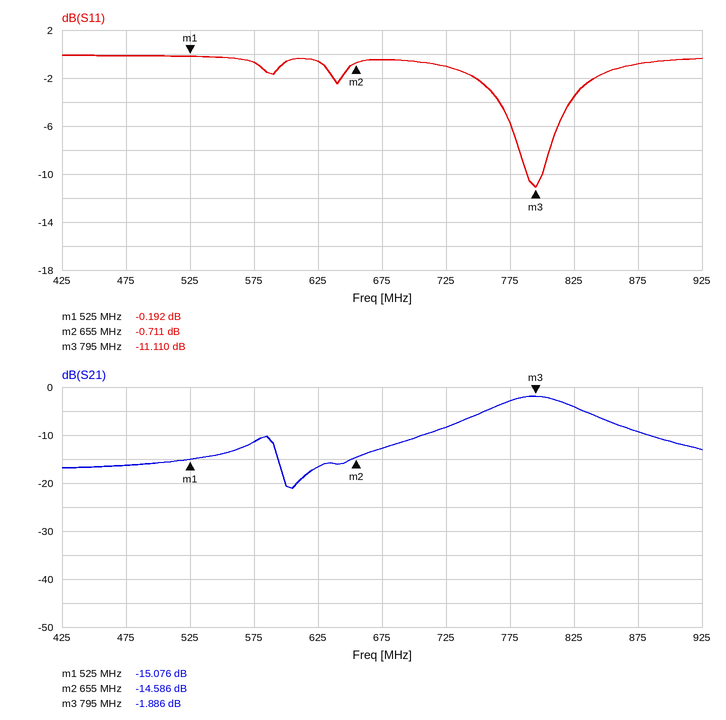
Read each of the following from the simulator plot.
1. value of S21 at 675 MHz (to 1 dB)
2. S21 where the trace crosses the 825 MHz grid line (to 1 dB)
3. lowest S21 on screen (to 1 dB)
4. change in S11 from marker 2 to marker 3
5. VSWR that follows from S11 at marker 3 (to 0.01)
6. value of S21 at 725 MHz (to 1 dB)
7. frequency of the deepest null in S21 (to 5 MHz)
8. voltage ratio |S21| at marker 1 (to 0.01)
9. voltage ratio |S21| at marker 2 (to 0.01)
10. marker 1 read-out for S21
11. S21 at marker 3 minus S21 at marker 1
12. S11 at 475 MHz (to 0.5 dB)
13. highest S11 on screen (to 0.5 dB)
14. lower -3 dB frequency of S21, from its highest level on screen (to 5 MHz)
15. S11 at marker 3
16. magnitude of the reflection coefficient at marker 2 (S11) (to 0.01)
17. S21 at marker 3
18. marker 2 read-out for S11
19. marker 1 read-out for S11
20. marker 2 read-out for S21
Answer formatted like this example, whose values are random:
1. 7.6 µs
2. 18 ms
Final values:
1. -13 dB
2. -4 dB
3. -21 dB
4. -10.399 dB
5. 1.77
6. -8 dB
7. 605 MHz
8. 0.18
9. 0.19
10. -15.076 dB
11. 13.190 dB
12. 0.0 dB
13. 0.0 dB
14. 755 MHz
15. -11.110 dB
16. 0.92
17. -1.886 dB
18. -0.711 dB
19. -0.192 dB
20. -14.586 dB
